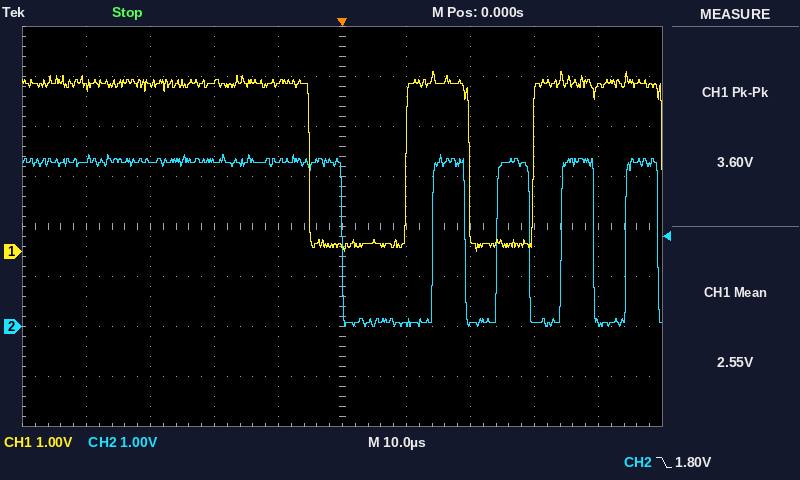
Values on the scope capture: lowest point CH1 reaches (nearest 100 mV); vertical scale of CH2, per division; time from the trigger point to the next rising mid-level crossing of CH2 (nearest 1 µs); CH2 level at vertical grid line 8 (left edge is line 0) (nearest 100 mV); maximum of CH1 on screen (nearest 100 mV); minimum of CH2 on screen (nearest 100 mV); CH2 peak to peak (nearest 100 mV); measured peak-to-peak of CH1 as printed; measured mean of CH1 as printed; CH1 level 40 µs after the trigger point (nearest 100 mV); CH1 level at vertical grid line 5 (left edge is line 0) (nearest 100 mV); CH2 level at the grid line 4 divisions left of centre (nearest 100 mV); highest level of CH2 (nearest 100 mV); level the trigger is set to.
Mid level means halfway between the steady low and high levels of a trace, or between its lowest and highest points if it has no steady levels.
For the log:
0.0 V
1 V
14 µs
100 mV
3.6 V
0.0 V
3.4 V
3.60 V
2.55 V
3.3 V
100 mV
3.4 V
3.4 V
1.80 V
